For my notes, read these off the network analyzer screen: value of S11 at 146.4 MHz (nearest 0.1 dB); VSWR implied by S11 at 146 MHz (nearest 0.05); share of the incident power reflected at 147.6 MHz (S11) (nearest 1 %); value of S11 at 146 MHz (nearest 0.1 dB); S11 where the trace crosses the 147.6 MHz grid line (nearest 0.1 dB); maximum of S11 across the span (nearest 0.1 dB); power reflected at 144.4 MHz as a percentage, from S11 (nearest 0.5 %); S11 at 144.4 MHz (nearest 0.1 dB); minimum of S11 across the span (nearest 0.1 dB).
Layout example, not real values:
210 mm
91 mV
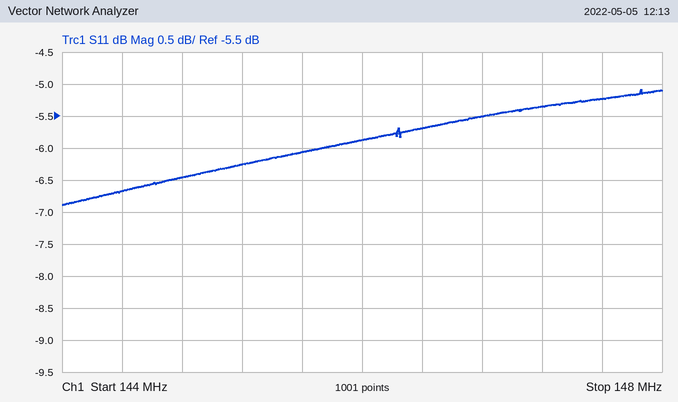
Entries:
-5.7 dB
3.05
30 %
-5.9 dB
-5.2 dB
-5.1 dB
21.5 %
-6.7 dB
-6.9 dB
